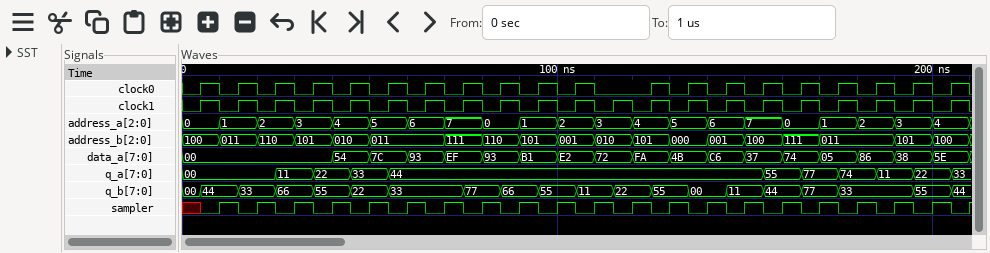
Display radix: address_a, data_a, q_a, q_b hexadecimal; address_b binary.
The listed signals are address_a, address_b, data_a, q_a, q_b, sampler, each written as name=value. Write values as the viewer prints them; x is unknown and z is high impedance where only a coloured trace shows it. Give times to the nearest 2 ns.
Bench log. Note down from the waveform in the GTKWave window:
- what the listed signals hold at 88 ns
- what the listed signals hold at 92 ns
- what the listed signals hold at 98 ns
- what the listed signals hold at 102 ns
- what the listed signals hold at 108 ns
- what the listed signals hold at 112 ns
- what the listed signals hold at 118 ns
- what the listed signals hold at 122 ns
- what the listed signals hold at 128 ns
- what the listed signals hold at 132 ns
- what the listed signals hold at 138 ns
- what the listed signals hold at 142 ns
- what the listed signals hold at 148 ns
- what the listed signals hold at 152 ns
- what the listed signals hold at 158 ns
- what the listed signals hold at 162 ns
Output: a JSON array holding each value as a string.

["address_a=0, address_b=110, data_a=93, q_a=44, q_b=66, sampler=0", "address_a=1, address_b=101, data_a=B1, q_a=44, q_b=66, sampler=1", "address_a=1, address_b=101, data_a=B1, q_a=44, q_b=55, sampler=0", "address_a=2, address_b=001, data_a=E2, q_a=44, q_b=55, sampler=1", "address_a=2, address_b=001, data_a=E2, q_a=44, q_b=11, sampler=0", "address_a=3, address_b=010, data_a=72, q_a=44, q_b=11, sampler=1", "address_a=3, address_b=010, data_a=72, q_a=44, q_b=22, sampler=0", "address_a=4, address_b=101, data_a=FA, q_a=44, q_b=22, sampler=1", "address_a=4, address_b=101, data_a=FA, q_a=44, q_b=55, sampler=0", "address_a=5, address_b=000, data_a=4B, q_a=44, q_b=55, sampler=1", "address_a=5, address_b=000, data_a=4B, q_a=44, q_b=00, sampler=0", "address_a=6, address_b=001, data_a=C6, q_a=44, q_b=00, sampler=1", "address_a=6, address_b=001, data_a=C6, q_a=44, q_b=11, sampler=0", "address_a=7, address_b=100, data_a=37, q_a=44, q_b=11, sampler=1", "address_a=7, address_b=100, data_a=37, q_a=55, q_b=44, sampler=0", "address_a=0, address_b=111, data_a=74, q_a=55, q_b=44, sampler=1"]
